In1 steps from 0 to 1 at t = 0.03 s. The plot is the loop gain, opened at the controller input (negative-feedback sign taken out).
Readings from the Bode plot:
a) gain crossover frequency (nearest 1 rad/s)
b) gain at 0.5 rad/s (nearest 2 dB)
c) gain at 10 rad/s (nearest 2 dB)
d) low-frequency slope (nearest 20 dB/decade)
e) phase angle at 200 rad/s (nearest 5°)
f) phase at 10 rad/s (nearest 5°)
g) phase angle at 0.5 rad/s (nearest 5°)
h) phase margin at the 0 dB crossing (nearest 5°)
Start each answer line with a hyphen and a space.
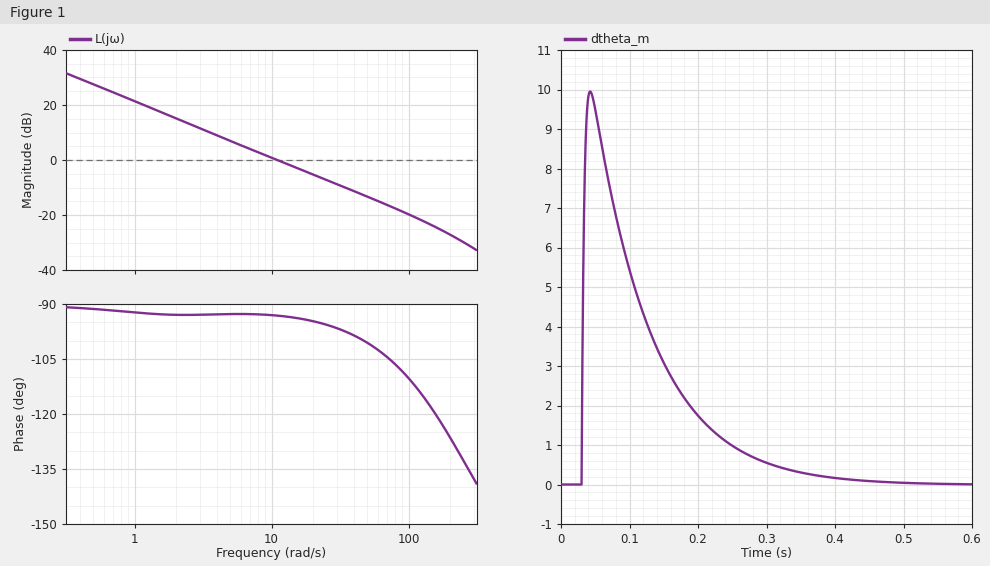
- 11 rad/s
- 28 dB
- 0 dB
- -20 dB/decade
- -125°
- -95°
- -90°
- 85°
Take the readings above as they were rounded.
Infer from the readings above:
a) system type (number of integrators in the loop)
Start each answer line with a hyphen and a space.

- 1
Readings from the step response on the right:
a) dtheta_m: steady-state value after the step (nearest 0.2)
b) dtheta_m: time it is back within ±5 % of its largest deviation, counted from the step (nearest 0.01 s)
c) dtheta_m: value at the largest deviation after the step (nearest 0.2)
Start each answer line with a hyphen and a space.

- 0.0
- 0.28 s
- 10.0
